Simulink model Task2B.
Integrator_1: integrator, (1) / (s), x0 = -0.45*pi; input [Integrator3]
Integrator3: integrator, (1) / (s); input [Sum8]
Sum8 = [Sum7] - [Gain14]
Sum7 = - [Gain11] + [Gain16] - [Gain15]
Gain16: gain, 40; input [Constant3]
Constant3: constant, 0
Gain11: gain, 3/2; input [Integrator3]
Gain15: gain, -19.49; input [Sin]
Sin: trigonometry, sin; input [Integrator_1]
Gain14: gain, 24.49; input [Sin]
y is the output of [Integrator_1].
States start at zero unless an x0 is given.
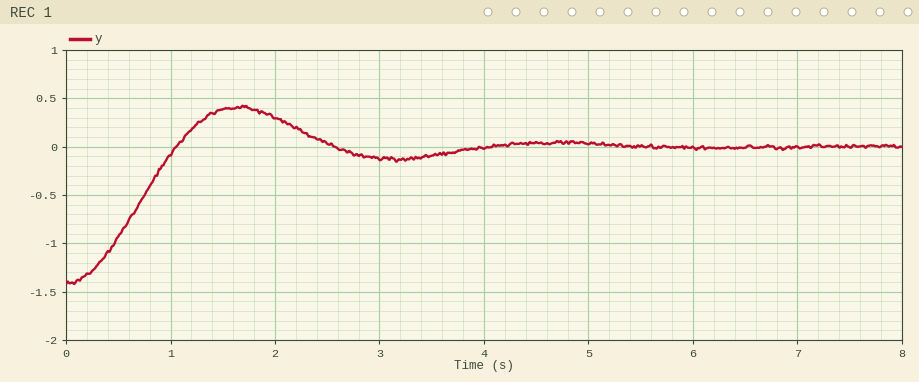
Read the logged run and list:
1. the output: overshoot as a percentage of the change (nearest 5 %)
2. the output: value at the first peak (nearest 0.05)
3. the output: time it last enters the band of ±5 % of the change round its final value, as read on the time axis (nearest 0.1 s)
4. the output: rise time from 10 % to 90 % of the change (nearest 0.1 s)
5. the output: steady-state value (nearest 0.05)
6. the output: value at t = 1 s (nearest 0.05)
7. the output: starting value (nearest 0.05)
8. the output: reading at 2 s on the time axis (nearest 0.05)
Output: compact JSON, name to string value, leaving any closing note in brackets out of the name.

{"the output: overshoot as a percentage of the change": "30 %", "the output: value at the first peak": "0.40", "the output: time it last enters the band of ±5 % of the change round its final value, as read on the time axis": "3.7 s", "the output: rise time from 10 % to 90 % of the change": "0.7 s", "the output: steady-state value": "0.00", "the output: value at t = 1 s": "-0.10", "the output: starting value": "-1.40", "the output: reading at 2 s on the time axis": "0.30"}
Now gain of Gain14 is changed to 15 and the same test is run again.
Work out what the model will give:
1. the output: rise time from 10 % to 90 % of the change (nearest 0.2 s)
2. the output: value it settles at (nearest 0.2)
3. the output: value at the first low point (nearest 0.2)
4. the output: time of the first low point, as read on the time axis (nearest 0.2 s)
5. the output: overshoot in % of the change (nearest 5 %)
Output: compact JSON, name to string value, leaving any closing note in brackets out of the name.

{"the output: rise time from 10 % to 90 % of the change": "0.8 s", "the output: value it settles at": "-3.2", "the output: value at the first low point": "-3.6", "the output: time of the first low point, as read on the time axis": "1.8 s", "the output: overshoot in % of the change": "25 %"}
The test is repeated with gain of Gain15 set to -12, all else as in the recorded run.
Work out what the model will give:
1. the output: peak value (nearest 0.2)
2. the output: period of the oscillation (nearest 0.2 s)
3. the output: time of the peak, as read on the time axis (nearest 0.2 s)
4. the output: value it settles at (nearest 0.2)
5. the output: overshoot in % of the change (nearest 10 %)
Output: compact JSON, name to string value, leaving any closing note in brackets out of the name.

{"the output: peak value": "0.6", "the output: period of the oscillation": "1.8 s", "the output: time of the peak, as read on the time axis": "1.0 s", "the output: value it settles at": "0.0", "the output: overshoot in % of the change": "50 %"}
